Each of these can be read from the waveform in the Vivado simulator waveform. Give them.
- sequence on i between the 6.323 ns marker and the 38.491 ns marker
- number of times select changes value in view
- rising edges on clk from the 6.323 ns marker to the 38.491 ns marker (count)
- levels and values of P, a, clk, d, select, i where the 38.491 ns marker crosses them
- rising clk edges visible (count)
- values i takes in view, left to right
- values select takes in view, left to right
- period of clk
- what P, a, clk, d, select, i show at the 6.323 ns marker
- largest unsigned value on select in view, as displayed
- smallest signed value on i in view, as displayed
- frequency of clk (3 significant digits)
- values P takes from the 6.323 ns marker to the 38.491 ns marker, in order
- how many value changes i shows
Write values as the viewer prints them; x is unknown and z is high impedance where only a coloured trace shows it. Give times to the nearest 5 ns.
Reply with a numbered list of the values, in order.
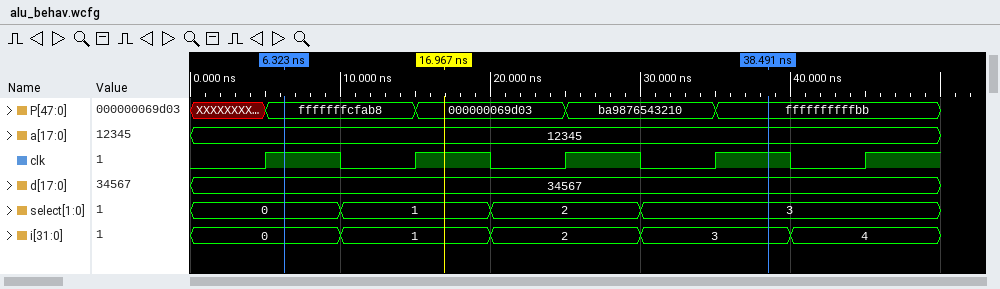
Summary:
1. 0, 1, 2, 3
2. 3
3. 3
4. P=ffffffffffbb, a=12345, clk=1, d=34567, select=3, i=3
5. 5
6. 0, 1, 2, 3, 4
7. 0, 1, 2, 3
8. 10 ns
9. P=fffffffcfab8, a=12345, clk=1, d=34567, select=0, i=0
10. 3
11. 0
12. 100 MHz
13. fffffffcfab8, 000000069d03, ba9876543210, ffffffffffbb
14. 4
